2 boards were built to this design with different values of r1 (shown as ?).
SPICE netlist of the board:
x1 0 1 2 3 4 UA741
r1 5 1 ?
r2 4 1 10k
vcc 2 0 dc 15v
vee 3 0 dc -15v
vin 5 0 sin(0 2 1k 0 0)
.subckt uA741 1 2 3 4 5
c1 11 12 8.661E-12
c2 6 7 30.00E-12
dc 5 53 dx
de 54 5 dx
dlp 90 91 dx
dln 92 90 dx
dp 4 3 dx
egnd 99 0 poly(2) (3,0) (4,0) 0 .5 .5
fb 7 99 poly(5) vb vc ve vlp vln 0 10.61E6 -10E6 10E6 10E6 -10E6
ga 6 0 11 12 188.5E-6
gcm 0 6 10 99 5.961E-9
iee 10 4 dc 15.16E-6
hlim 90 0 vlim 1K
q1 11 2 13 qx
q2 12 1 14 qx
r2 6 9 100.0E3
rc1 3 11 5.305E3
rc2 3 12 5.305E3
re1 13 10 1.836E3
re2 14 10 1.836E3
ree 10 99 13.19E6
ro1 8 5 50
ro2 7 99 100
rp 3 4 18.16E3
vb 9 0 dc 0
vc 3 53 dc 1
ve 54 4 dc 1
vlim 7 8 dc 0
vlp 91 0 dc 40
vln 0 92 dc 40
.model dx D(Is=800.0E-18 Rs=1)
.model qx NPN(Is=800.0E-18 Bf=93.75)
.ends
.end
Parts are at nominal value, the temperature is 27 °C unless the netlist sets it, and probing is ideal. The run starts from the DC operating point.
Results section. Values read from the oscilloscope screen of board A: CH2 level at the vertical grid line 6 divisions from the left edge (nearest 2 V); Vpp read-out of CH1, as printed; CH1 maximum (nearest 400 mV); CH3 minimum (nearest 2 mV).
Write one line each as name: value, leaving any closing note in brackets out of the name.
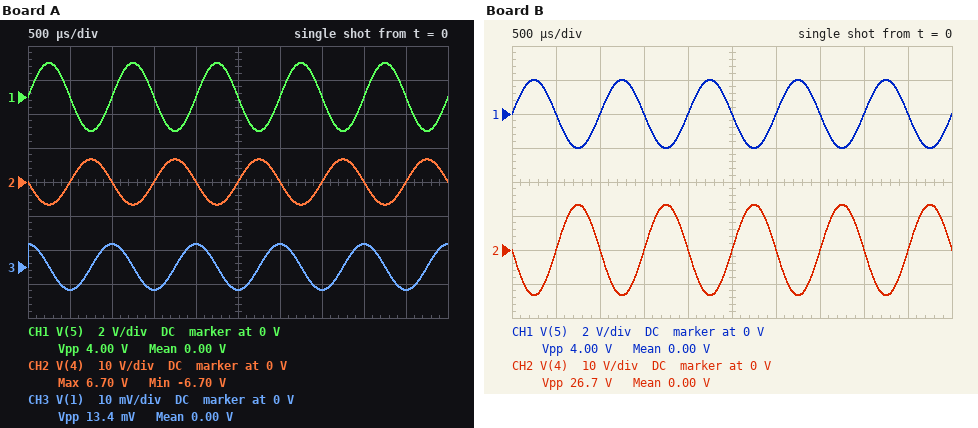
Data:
CH2 level at the vertical grid line 6 divisions from the left edge: 0 V
Vpp read-out of CH1, as printed: 4.00 V
CH1 maximum: 2.0 V
CH3 minimum: -6 mV
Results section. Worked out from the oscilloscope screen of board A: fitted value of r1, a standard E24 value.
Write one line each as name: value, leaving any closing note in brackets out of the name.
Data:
fitted value of r1, a standard E24 value: 3 kΩ
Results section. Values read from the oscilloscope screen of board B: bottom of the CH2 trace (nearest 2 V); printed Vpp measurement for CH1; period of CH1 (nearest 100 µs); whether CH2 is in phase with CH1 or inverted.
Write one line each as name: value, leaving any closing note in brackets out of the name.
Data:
bottom of the CH2 trace: -14 V
printed Vpp measurement for CH1: 4.00 V
period of CH1: 1.0 ms
whether CH2 is in phase with CH1 or inverted: inverted
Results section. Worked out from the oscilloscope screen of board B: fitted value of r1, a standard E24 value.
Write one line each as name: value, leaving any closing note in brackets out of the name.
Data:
fitted value of r1, a standard E24 value: 1.5 kΩ
